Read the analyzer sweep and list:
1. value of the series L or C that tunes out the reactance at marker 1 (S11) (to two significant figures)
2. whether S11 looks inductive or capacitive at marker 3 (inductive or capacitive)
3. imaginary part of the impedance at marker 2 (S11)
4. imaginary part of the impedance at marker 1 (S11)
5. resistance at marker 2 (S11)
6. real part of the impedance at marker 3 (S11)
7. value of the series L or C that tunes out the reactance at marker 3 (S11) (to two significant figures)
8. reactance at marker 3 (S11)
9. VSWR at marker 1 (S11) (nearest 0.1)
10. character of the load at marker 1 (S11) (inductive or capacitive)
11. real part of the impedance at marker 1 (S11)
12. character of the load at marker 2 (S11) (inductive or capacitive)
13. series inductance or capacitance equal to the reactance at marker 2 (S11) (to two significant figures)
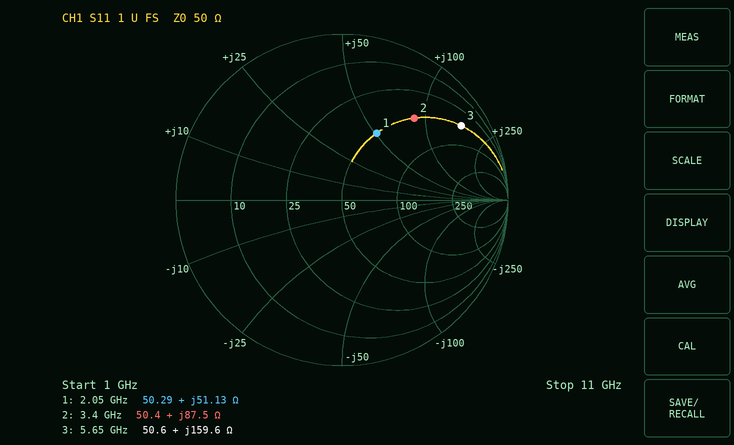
1.5 pF
inductive
+87.5 Ω
+51.13 Ω
50.4 Ω
50.6 Ω
180 fF
+159.6 Ω
2.7
inductive
50.29 Ω
inductive
4.1 nH
